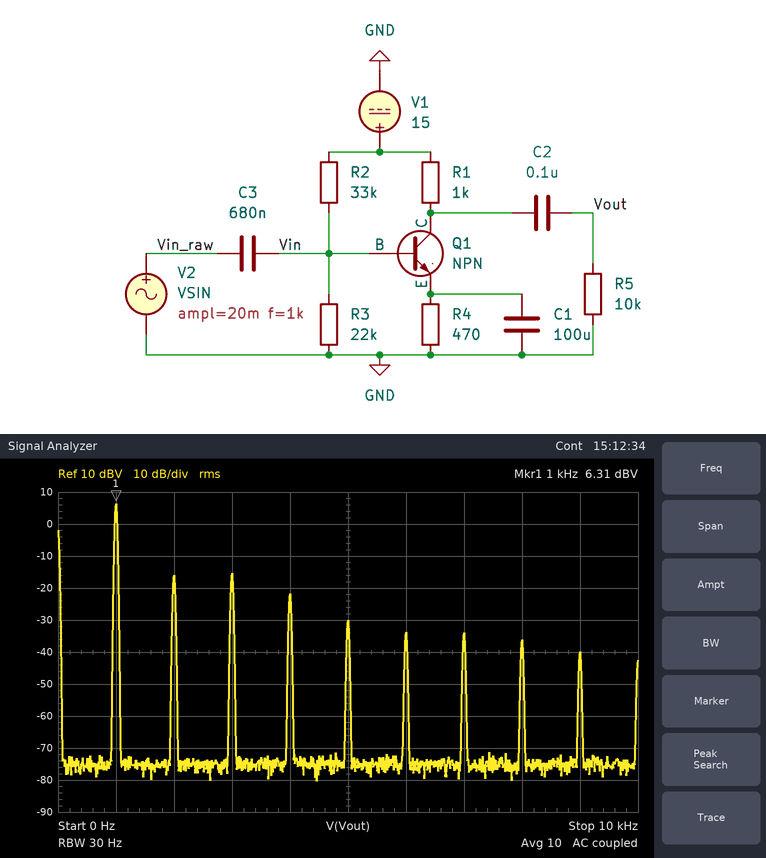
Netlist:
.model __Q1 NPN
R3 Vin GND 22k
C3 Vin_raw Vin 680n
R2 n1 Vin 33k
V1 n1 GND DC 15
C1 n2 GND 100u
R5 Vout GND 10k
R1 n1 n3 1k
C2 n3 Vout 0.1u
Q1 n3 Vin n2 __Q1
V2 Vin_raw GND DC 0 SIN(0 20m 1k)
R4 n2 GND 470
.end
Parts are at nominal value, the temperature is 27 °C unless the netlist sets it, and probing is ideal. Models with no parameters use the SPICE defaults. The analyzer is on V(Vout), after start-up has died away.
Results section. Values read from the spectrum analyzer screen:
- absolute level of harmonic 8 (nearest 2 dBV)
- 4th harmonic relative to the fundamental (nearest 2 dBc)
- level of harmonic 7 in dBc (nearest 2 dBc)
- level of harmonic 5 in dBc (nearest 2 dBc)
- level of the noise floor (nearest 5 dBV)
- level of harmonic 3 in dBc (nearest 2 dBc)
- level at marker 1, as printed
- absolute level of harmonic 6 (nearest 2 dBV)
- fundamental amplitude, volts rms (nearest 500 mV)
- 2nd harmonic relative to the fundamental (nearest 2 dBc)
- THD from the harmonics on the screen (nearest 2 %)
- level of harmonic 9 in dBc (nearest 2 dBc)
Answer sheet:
-36 dBV
-28 dBc
-40 dBc
-36 dBc
-75 dBV
-22 dBc
6.31 dBV
-34 dBV
2.0 V
-22 dBc
12 %
-46 dBc
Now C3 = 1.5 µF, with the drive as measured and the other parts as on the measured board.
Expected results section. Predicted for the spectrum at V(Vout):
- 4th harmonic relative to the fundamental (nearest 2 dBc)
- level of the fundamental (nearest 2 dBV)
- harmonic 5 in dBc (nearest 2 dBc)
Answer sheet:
-26 dBc
8 dBV
-34 dBc
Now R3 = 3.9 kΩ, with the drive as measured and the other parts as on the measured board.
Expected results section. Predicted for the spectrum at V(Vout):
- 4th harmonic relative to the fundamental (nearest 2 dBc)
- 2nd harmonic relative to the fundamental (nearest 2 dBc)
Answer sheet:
-52 dBc
-14 dBc
